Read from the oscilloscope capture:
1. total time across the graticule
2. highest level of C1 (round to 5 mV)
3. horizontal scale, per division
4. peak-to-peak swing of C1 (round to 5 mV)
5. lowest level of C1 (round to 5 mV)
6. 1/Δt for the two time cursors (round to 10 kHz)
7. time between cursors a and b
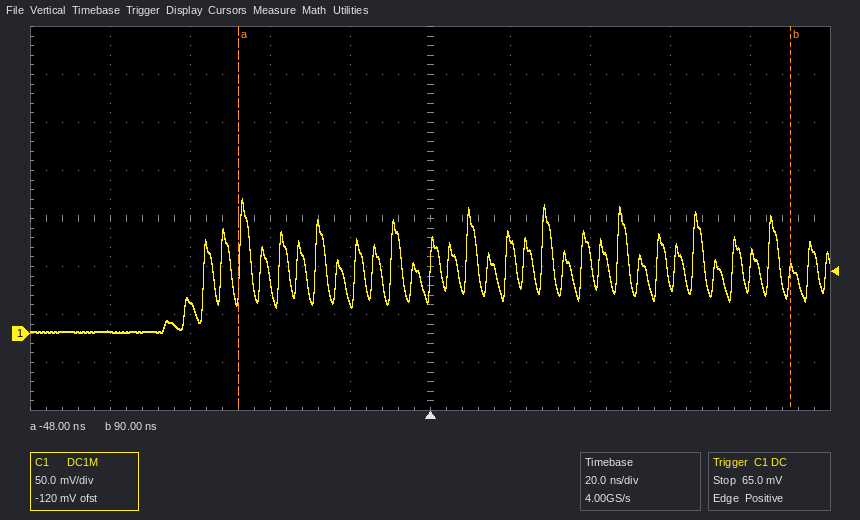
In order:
200 ns
140 mV
20 ns
140 mV
0 mV
7.25 MHz
138 ns
